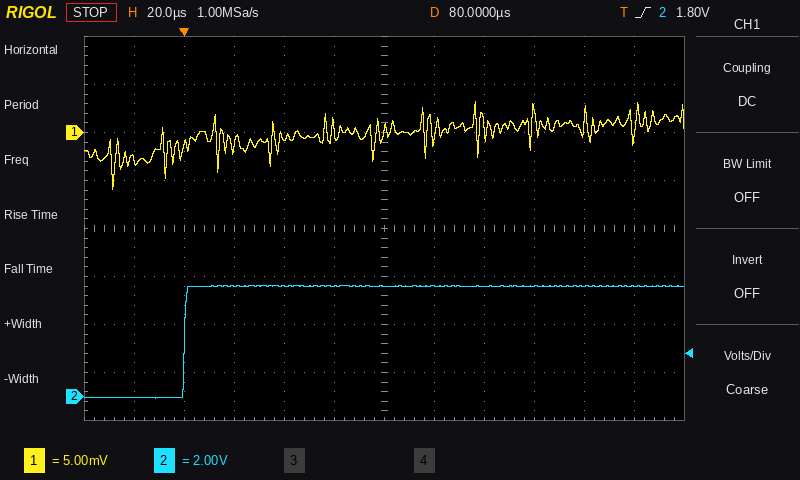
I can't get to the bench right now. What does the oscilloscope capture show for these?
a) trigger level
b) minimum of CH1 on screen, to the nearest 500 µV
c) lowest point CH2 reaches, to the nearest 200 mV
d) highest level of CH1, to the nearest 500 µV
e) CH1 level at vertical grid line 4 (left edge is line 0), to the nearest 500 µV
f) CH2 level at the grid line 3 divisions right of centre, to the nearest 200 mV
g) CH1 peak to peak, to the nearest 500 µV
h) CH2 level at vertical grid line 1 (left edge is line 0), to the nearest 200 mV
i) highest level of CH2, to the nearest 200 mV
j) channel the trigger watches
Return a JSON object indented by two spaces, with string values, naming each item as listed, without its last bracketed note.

{
  "trigger level": "1.80 V",
  "minimum of CH1 on screen, to the nearest 500 µV": "-6.0 mV",
  "lowest point CH2 reaches, to the nearest 200 mV": "0.0 V",
  "highest level of CH1, to the nearest 500 µV": "3.0 mV",
  "CH1 level at vertical grid line 4 (left edge is line 0), to the nearest 500 µV": "-500 µV",
  "CH2 level at the grid line 3 divisions right of centre, to the nearest 200 mV": "4.6 V",
  "CH1 peak to peak, to the nearest 500 µV": "9.0 mV",
  "CH2 level at vertical grid line 1 (left edge is line 0), to the nearest 200 mV": "0.0 V",
  "highest level of CH2, to the nearest 200 mV": "4.6 V",
  "channel the trigger watches": "CH2"
}
